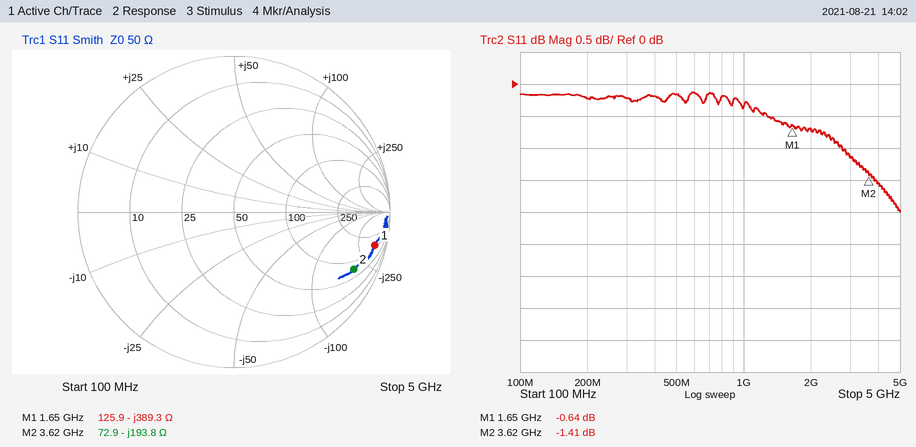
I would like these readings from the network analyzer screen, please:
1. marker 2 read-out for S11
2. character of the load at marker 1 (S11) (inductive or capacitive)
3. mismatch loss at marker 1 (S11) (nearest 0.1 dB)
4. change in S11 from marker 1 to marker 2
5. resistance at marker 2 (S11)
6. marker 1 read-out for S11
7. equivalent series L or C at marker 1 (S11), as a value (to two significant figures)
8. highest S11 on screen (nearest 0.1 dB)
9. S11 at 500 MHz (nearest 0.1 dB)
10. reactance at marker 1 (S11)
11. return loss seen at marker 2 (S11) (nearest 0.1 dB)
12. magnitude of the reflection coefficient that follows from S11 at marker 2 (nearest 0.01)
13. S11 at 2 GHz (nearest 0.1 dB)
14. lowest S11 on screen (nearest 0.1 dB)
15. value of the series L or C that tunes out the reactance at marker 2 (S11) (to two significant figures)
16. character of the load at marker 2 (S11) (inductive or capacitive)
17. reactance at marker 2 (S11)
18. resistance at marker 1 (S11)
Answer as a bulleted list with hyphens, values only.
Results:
- -1.41 dB
- capacitive
- 8.6 dB
- -0.77 dB
- 72.9 Ω
- -0.64 dB
- 250 fF
- -0.1 dB
- -0.2 dB
- -389.3 Ω
- 1.4 dB
- 0.85
- -0.7 dB
- -2.0 dB
- 8.5 nH
- capacitive
- -193.8 Ω
- 125.9 Ω
